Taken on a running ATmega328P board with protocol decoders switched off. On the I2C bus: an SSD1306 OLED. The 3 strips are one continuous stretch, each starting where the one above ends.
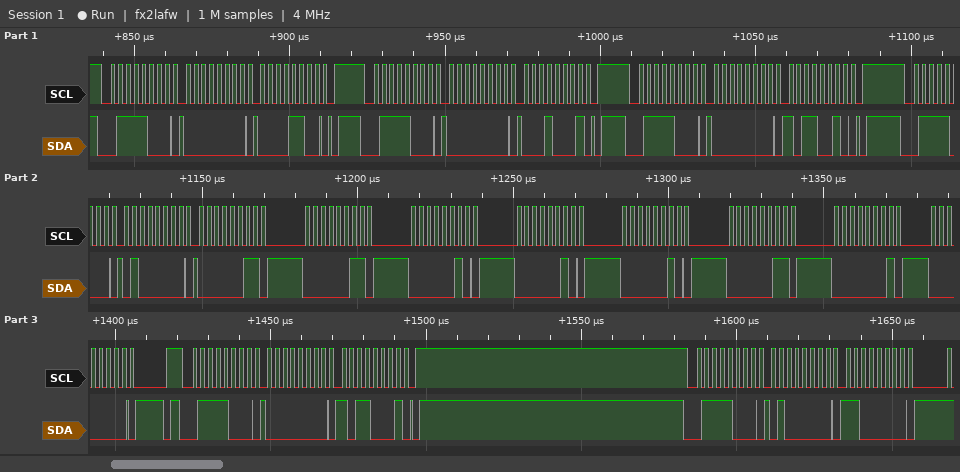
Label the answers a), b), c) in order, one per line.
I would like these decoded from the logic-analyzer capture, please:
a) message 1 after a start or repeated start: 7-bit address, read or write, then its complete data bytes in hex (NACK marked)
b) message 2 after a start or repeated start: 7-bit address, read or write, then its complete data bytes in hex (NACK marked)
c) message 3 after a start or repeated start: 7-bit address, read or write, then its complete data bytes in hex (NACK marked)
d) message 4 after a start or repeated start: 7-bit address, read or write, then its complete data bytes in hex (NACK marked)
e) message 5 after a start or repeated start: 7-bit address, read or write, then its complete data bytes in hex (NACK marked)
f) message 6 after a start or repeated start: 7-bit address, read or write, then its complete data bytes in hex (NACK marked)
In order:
a) 0x3C write: 00 0C
b) 0x3C write: 00 11
c) 0x3C write: 00 B2
d) 0x3C write: 40 03 03 02 02 02 03 01 00
e) 0x3C write: 00 B1
f) 0x3C write: 40 C0
